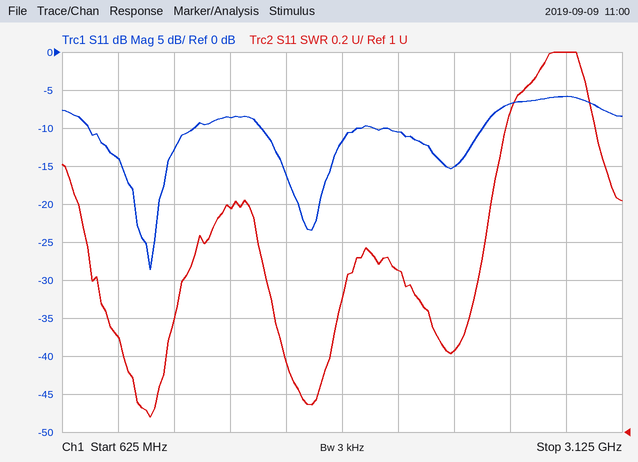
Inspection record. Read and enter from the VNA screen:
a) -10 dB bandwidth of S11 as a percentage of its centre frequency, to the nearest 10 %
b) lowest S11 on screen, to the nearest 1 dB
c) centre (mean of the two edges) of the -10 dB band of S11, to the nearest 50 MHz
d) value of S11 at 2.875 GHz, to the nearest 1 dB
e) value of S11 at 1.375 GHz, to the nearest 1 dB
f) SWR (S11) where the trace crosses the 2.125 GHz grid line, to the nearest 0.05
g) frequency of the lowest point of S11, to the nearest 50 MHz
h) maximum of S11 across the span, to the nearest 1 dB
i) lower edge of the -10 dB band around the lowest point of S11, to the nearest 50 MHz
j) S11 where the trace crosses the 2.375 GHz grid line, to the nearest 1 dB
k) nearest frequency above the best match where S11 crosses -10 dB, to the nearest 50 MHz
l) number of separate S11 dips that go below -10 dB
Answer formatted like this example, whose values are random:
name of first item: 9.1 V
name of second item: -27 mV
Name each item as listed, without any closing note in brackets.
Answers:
-10 dB bandwidth of S11 as a percentage of its centre frequency, to the nearest 10 %: 50 %
lowest S11 on screen, to the nearest 1 dB: -29 dB
centre (mean of the two edges) of the -10 dB band of S11, to the nearest 50 MHz: 1.00 GHz
value of S11 at 2.875 GHz, to the nearest 1 dB: -6 dB
value of S11 at 1.375 GHz, to the nearest 1 dB: -9 dB
SWR (S11) where the trace crosses the 2.125 GHz grid line, to the nearest 0.05: 1.85
frequency of the lowest point of S11, to the nearest 50 MHz: 1.00 GHz
maximum of S11 across the span, to the nearest 1 dB: -6 dB
lower edge of the -10 dB band around the lowest point of S11, to the nearest 50 MHz: 750 MHz
S11 where the trace crosses the 2.375 GHz grid line, to the nearest 1 dB: -15 dB
nearest frequency above the best match where S11 crosses -10 dB, to the nearest 50 MHz: 1.20 GHz
number of separate S11 dips that go below -10 dB: 3
